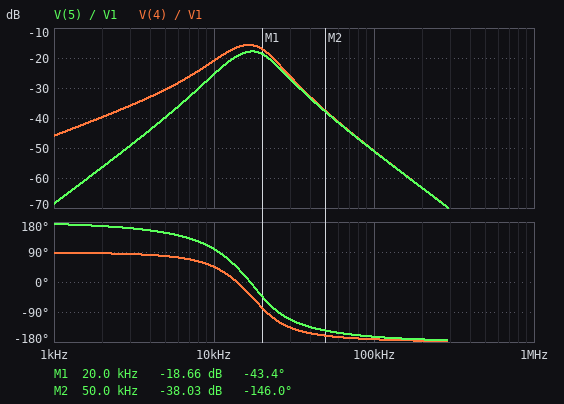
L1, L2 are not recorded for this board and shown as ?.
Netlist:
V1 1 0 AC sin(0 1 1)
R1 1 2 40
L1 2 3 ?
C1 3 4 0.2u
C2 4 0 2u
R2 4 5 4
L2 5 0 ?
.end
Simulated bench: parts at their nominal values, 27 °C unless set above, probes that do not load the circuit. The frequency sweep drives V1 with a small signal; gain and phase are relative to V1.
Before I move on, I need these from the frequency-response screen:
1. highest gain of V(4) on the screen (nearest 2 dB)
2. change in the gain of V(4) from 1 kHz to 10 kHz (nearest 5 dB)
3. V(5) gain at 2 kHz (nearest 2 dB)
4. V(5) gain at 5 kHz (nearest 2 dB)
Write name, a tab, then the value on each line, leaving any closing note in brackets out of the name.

highest gain of V(4) on the screen	-16 dB
change in the gain of V(4) from 1 kHz to 10 kHz	25 dB
V(5) gain at 2 kHz	-56 dB
V(5) gain at 5 kHz	-40 dB
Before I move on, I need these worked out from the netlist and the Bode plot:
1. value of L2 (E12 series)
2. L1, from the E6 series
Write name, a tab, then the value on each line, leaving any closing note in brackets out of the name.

value of L2	47 µH
L1, from the E6 series	470 µH
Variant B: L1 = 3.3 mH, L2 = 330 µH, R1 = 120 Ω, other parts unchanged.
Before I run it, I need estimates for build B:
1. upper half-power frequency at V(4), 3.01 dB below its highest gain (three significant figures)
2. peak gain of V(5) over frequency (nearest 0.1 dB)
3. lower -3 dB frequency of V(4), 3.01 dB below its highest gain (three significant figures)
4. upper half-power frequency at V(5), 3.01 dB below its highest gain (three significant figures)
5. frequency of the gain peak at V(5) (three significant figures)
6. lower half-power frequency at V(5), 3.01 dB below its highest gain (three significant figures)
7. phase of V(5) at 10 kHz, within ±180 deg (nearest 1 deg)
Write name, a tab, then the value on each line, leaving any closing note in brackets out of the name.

upper half-power frequency at V(4), 3.01 dB below its highest gain	7.64 kHz
peak gain of V(5) over frequency	-11.8 dB
lower -3 dB frequency of V(4), 3.01 dB below its highest gain	5.14 kHz
upper half-power frequency at V(5), 3.01 dB below its highest gain	7.67 kHz
frequency of the gain peak at V(5)	6.35 kHz
lower half-power frequency at V(5), 3.01 dB below its highest gain	5.18 kHz
phase of V(5) at 10 kHz, within ±180 deg	-116 deg
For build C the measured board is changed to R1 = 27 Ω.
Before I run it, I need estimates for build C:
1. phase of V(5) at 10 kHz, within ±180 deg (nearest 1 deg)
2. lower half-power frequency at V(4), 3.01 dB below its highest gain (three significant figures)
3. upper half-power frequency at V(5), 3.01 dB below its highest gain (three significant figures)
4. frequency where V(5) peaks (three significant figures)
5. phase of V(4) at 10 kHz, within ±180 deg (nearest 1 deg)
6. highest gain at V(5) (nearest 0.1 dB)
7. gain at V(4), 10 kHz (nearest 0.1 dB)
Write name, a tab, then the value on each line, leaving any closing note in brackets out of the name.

phase of V(5) at 10 kHz, within ±180 deg	108 deg
lower half-power frequency at V(4), 3.01 dB below its highest gain	12.5 kHz
upper half-power frequency at V(5), 3.01 dB below its highest gain	21.9 kHz
frequency where V(5) peaks	17.5 kHz
phase of V(4) at 10 kHz, within ±180 deg	54 deg
highest gain at V(5)	-14.8 dB
gain at V(4), 10 kHz	-19.8 dB
